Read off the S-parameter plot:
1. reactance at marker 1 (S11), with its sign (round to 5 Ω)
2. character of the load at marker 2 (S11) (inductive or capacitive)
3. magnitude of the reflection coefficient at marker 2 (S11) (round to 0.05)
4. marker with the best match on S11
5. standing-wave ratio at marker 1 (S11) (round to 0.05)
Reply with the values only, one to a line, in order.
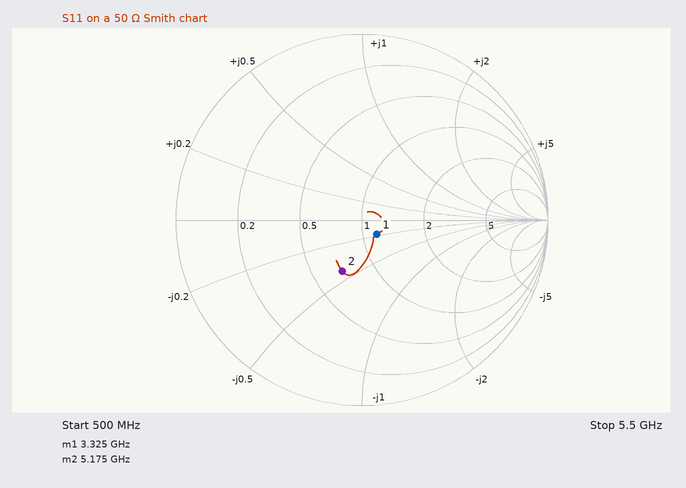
-10 Ω
capacitive
0.30
marker 1
1.25
